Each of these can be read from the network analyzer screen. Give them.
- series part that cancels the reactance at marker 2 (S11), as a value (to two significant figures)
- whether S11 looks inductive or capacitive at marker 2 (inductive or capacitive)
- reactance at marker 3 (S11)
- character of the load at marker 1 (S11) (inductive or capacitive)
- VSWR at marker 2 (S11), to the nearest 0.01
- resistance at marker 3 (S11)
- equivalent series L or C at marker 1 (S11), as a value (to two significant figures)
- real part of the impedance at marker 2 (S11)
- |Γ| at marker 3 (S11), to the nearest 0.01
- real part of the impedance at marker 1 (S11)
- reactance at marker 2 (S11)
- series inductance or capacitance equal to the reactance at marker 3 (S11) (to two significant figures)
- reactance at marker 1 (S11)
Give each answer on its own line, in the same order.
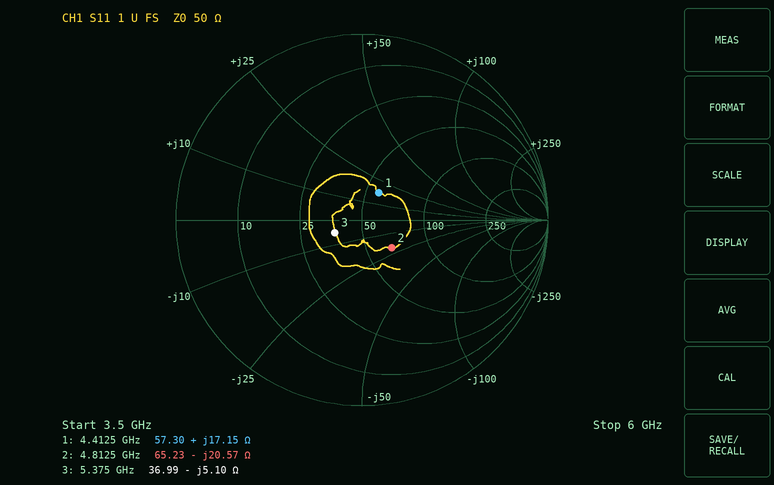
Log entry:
680 pH
capacitive
-5.10 Ω
inductive
1.56
36.99 Ω
620 pH
65.23 Ω
0.16
57.30 Ω
-20.57 Ω
5.8 pF
+17.15 Ω
